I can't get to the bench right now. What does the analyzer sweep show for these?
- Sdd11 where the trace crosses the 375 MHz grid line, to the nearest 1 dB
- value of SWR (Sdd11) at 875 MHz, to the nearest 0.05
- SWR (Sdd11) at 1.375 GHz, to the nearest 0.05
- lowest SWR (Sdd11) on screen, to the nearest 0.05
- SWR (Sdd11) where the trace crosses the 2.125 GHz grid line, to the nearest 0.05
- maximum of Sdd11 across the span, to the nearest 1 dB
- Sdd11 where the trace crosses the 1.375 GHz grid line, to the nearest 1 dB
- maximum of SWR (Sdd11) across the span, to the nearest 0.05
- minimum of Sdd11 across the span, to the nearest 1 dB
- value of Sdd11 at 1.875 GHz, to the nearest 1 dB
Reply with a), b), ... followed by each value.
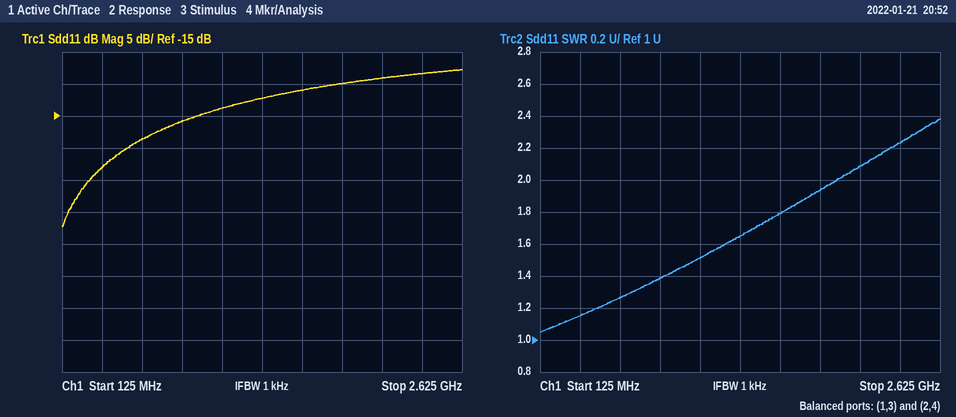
a) -23 dB
b) 1.40
c) 1.65
d) 1.05
e) 2.10
f) -8 dB
g) -12 dB
h) 2.40
i) -32 dB
j) -10 dB
